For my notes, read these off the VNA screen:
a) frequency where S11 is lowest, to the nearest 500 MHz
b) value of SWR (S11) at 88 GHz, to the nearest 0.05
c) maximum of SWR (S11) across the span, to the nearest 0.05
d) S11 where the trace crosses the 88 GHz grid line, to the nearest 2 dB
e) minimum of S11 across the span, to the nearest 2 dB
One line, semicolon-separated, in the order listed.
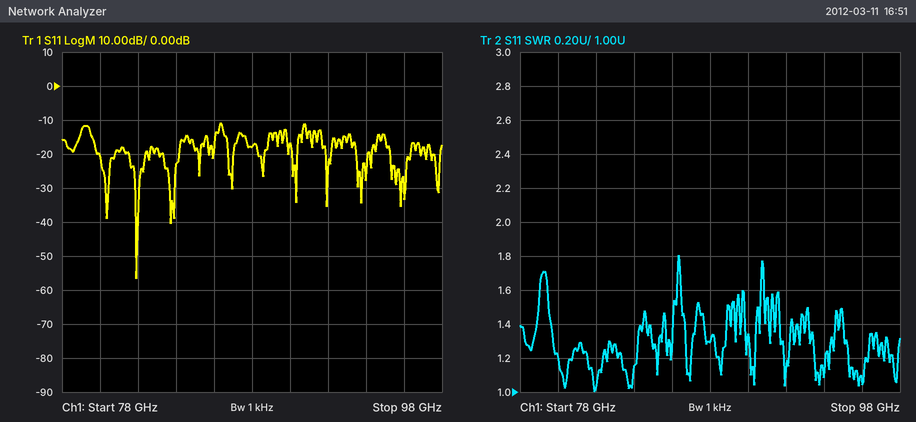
82.0 GHz; 1.30; 1.80; -18 dB; -56 dB
